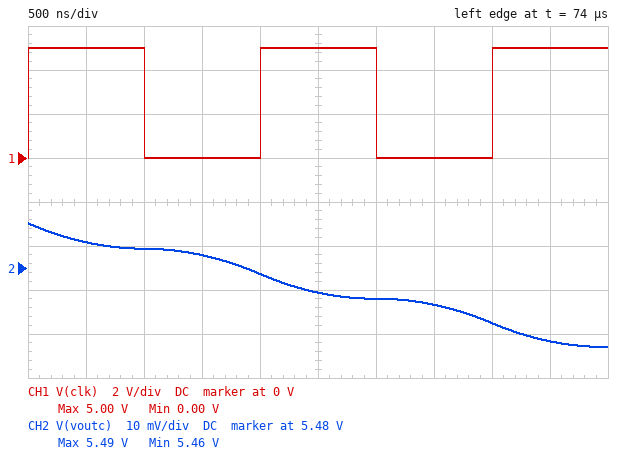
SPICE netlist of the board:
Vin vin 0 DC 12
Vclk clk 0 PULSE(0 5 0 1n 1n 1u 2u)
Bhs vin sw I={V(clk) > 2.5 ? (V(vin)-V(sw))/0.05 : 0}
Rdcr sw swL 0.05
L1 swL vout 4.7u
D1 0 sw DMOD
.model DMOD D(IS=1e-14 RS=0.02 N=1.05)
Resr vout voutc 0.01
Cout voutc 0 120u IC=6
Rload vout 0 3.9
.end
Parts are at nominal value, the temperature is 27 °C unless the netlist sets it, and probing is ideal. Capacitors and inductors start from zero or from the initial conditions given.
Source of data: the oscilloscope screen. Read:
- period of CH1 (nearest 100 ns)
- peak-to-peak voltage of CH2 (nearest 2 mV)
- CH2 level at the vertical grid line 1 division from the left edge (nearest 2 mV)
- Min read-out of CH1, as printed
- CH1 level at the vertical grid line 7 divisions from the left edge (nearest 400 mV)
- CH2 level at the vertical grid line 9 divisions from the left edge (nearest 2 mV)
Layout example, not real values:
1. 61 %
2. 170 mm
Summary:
1. 2.0 µs
2. 28 mV
3. 5.486 V
4. 0.00 V
5. 0 V
6. 5.464 V
